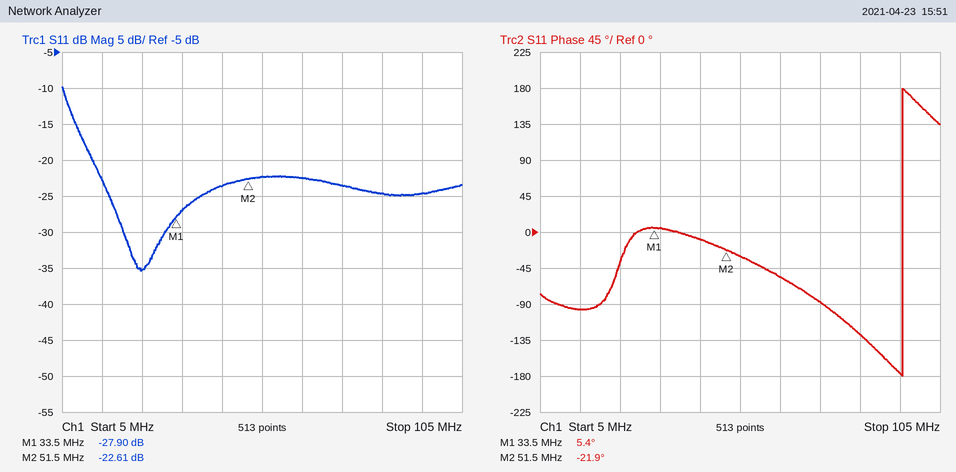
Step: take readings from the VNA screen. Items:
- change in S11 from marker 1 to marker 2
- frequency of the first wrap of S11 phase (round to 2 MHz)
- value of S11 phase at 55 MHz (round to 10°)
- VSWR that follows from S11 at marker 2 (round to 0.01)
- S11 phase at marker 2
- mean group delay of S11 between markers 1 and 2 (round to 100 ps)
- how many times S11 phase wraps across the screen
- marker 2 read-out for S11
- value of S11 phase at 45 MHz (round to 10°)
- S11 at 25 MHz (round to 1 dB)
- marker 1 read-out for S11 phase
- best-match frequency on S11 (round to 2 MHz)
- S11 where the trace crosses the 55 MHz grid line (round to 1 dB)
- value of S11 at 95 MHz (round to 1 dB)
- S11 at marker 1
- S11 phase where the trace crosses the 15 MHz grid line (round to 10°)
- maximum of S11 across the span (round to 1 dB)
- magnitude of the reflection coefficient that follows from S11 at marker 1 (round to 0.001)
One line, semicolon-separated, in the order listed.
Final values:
5.29 dB; 96 MHz; -30°; 1.16; -21.9°; 4.2 ns; 1; -22.61 dB; -10°; -35 dB; 5.4°; 24 MHz; -22 dB; -25 dB; -27.90 dB; -100°; -10 dB; 0.040
